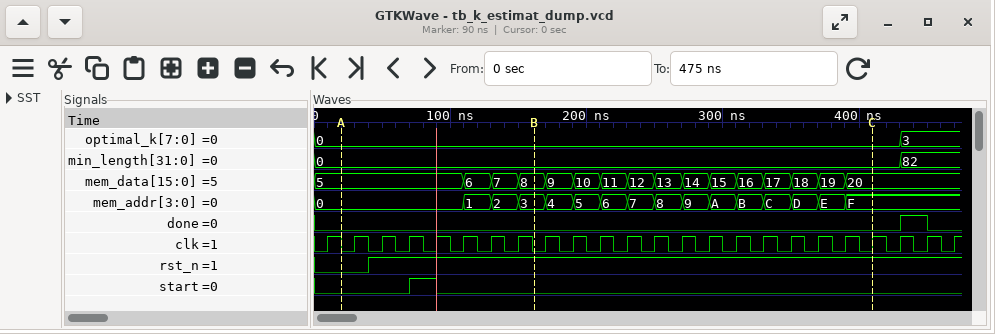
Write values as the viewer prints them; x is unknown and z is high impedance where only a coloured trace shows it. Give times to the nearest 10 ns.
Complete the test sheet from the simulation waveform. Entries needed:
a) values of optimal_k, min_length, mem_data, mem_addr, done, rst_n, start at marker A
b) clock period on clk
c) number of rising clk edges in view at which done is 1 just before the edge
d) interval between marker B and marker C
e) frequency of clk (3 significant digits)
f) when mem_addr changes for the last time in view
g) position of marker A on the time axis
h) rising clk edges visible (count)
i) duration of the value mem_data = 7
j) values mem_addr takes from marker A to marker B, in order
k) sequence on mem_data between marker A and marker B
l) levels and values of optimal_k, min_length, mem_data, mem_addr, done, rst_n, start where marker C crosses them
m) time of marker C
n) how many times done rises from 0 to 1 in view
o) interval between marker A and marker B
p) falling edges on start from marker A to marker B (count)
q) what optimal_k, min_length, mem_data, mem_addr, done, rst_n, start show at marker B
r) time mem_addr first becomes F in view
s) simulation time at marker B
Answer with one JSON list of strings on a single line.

["optimal_k=0, min_length=0, mem_data=5, mem_addr=0, done=0, rst_n=0, start=0", "20 ns", "1", "250 ns", "50.0 MHz", "390 ns", "20 ns", "24", "20 ns", "0, 1, 2, 3", "5, 6, 7, 8", "optimal_k=0, min_length=0, mem_data=20, mem_addr=F, done=0, rst_n=1, start=0", "410 ns", "1", "140 ns", "1", "optimal_k=0, min_length=0, mem_data=8, mem_addr=3, done=0, rst_n=1, start=0", "390 ns", "160 ns"]
